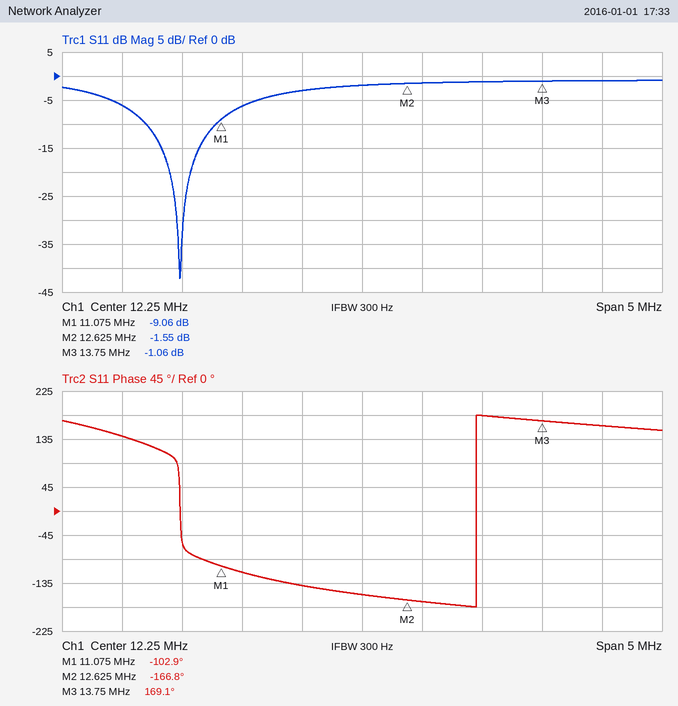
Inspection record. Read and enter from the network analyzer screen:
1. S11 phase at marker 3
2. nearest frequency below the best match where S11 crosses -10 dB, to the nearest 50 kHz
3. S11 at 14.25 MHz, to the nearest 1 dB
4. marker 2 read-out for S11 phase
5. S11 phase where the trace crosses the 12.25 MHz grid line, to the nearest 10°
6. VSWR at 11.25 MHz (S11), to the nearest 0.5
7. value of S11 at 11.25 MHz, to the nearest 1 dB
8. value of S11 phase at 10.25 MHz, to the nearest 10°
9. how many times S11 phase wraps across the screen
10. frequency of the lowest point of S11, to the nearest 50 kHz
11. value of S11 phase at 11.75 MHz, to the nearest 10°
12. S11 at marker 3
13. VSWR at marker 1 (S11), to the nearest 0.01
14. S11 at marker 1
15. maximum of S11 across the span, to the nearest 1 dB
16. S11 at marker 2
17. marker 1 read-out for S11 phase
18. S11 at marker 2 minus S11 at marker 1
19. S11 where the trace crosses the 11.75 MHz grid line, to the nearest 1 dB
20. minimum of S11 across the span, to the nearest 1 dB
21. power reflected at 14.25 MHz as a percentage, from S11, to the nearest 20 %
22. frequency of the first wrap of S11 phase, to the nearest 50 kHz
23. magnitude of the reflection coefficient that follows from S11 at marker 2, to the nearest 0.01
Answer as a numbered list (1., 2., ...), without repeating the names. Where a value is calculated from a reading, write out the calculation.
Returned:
1. 169.1°
2. 10.45 MHz
3. -1 dB
4. -166.8°
5. -160°
6. |Γ| = 10^(-6/20) = 0.5012; VSWR = (1 + 0.5012)/(1 − 0.5012) ≈ 3.0
7. -6 dB
8. 140°
9. 1
10. 10.75 MHz
11. -140°
12. -1.06 dB
13. (1 + 0.3524)/(1 − 0.3524) ≈ 2.09
14. -9.06 dB
15. -1 dB
16. -1.55 dB
17. -102.9°
18. -1.55 − (-9.06) = 7.51 dB
19. -3 dB
20. -42 dB
21. 10^(-1/10) ≈ 79.4 %, so 80 % to the nearest 20 %
22. 13.20 MHz
23. 10^(-1.55/20) ≈ 0.84
